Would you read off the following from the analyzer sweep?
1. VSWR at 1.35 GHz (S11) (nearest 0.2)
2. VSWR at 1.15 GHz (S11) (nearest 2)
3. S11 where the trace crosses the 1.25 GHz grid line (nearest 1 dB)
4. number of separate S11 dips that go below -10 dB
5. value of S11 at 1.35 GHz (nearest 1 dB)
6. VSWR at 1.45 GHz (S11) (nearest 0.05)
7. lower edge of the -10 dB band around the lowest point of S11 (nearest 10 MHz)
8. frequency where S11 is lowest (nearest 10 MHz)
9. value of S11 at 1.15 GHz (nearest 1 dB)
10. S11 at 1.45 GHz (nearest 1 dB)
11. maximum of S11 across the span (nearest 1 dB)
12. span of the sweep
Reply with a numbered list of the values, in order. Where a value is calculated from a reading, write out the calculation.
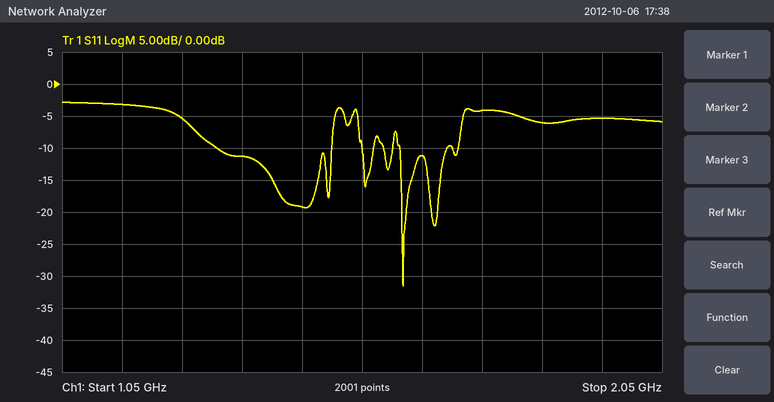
1. |Γ| = 10^(-11/20) = 0.2818; VSWR = (1 + 0.2818)/(1 − 0.2818) ≈ 1.8
2. |Γ| = 10^(-3/20) = 0.7079; VSWR = (1 + 0.7079)/(1 − 0.7079) ≈ 6
3. -5 dB
4. 6
5. -11 dB
6. |Γ| = 10^(-19/20) = 0.1122; VSWR = (1 + 0.1122)/(1 − 0.1122) ≈ 1.25
7. 1.61 GHz
8. 1.62 GHz
9. -3 dB
10. -19 dB
11. -3 dB
12. 1 GHz
